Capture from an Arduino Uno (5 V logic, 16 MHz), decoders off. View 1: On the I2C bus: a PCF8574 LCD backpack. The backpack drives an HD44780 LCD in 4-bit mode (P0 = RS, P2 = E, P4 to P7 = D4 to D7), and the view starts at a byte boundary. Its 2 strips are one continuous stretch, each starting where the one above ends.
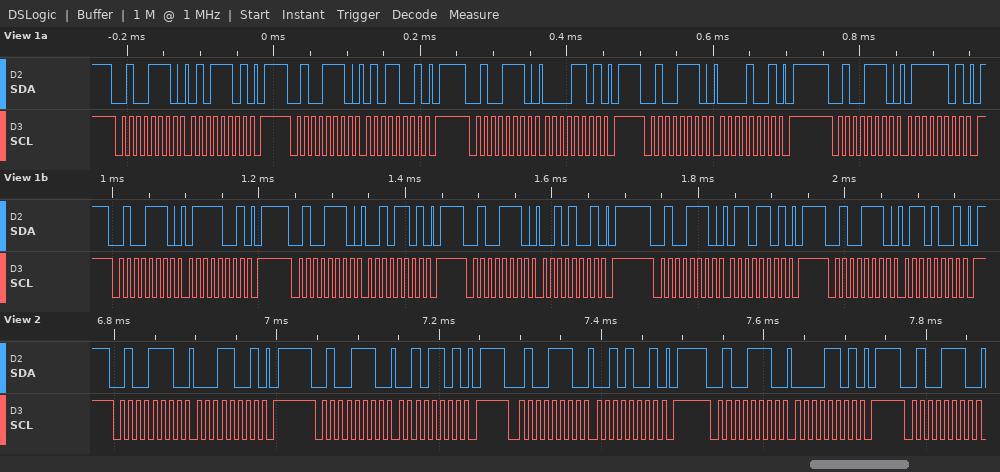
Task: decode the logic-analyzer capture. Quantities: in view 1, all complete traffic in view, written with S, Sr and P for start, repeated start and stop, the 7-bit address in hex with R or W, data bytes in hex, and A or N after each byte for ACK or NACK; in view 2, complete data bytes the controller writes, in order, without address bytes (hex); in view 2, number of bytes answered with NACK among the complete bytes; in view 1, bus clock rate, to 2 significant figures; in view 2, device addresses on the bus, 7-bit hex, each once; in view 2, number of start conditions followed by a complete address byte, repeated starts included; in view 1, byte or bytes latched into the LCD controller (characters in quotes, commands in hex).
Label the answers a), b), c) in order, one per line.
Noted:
a) S 27W A 5D A P S 27W A 59 A P S 27W A 0D A P S 27W A 09 A P S 27W A 7D A P S 27W A 79 A P S 27W A 2D A P S 27W A 29 A P S 27W A 6D A P S 27W A 69 A P
b) 19 2D 29 0D
c) 0
d) 100 kHz
e) 0x27
f) 5
g) 'P' 'r'
